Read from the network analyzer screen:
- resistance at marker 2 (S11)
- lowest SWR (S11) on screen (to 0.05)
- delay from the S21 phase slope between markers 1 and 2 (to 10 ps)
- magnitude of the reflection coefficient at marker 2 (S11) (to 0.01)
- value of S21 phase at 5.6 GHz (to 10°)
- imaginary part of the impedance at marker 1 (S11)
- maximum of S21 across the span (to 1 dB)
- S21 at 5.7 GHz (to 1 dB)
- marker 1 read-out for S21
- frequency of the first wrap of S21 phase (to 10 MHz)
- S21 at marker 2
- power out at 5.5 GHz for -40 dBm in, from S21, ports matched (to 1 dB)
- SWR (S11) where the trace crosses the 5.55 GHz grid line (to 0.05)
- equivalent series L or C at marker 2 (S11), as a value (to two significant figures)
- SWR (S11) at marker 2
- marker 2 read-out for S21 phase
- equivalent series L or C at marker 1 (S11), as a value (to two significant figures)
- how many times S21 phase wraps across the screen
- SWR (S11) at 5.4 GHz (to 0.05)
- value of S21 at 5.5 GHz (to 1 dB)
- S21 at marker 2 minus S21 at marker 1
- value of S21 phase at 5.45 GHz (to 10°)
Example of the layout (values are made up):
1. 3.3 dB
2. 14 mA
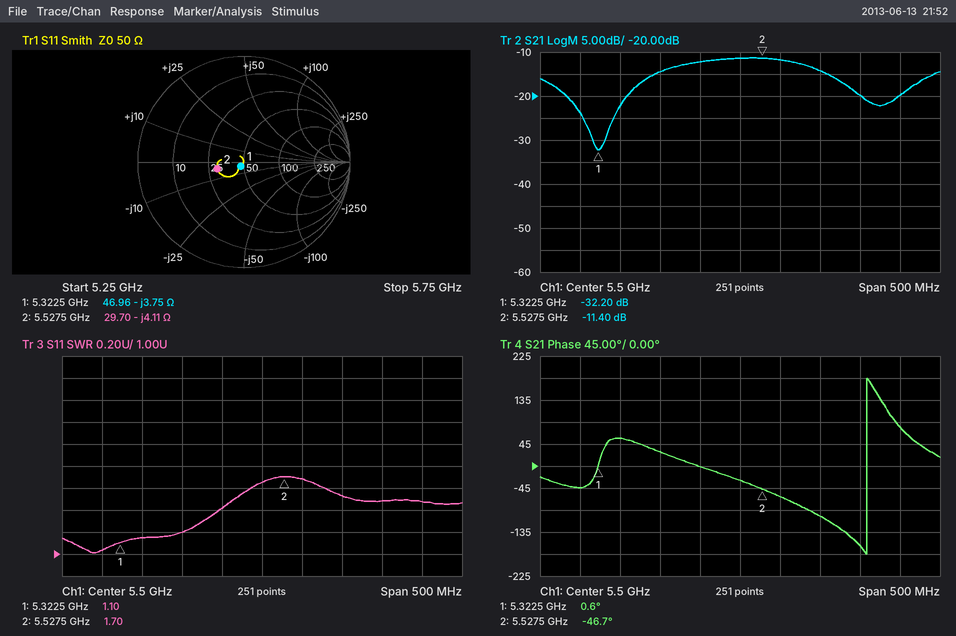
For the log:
1. 29.70 Ω
2. 1.00
3. 640 ps
4. 0.26
5. -100°
6. -3.75 Ω
7. -11 dB
8. -20 dB
9. -32.20 dB
10. 5.66 GHz
11. -11.40 dB
12. -51 dBm
13. 1.70
14. 7.0 pF
15. 1.70
16. -46.7°
17. 8.0 pF
18. 1
19. 1.20
20. -11 dB
21. 20.80 dB
22. 0°
